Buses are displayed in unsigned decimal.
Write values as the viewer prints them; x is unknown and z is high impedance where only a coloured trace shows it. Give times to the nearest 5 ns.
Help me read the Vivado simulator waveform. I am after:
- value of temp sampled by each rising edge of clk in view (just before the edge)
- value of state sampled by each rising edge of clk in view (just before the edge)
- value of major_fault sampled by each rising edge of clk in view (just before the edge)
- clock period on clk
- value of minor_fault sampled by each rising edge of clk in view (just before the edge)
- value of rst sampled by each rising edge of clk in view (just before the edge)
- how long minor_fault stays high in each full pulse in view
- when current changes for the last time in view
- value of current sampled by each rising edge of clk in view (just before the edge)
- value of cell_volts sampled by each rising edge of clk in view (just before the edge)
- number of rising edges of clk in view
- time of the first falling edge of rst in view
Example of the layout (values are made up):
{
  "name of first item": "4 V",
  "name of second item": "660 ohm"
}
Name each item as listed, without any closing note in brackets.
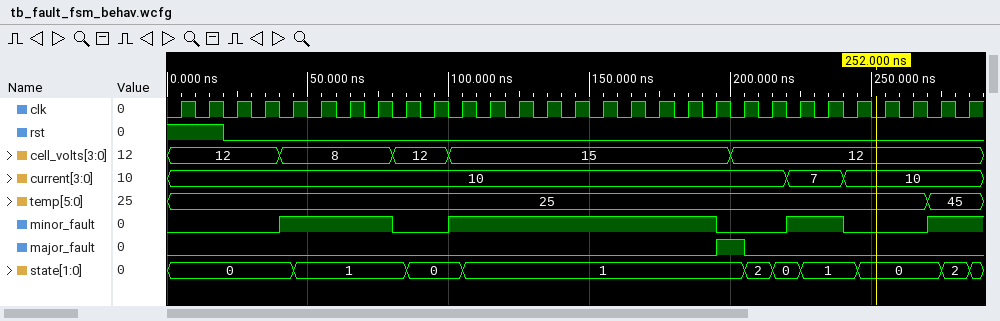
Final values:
{
  "value of temp sampled by each rising edge of clk in view": "25, 25, 25, 25, 25, 25, 25, 25, 25, 25, 25, 25, 25, 25, 25, 25, 25, 25, 25, 25, 25, 25, 25, 25, 25, 25, 25, 45, 45",
  "value of state sampled by each rising edge of clk in view": "0, 0, 0, 0, 0, 1, 1, 1, 1, 0, 0, 1, 1, 1, 1, 1, 1, 1, 1, 1, 1, 2, 0, 1, 1, 0, 0, 0, 2",
  "value of major_fault sampled by each rising edge of clk in view": "0 0 0 0 0 0 0 0 0 0 0 0 0 0 0 0 0 0 0 0 1 0 0 0 0 0 0 0 0",
  "clock period on clk": "10 ns",
  "value of minor_fault sampled by each rising edge of clk in view": "0 0 0 0 1 1 1 1 0 0 1 1 1 1 1 1 1 1 1 1 0 0 1 1 0 0 0 1 1",
  "value of rst sampled by each rising edge of clk in view": "1 1 0 0 0 0 0 0 0 0 0 0 0 0 0 0 0 0 0 0 0 0 0 0 0 0 0 0 0",
  "how long minor_fault stays high in each full pulse in view": "40 ns, 95 ns, 20 ns",
  "when current changes for the last time in view": "240 ns",
  "value of current sampled by each rising edge of clk in view": "10, 10, 10, 10, 10, 10, 10, 10, 10, 10, 10, 10, 10, 10, 10, 10, 10, 10, 10, 10, 10, 10, 7, 7, 10, 10, 10, 10, 10",
  "value of cell_volts sampled by each rising edge of clk in view": "12, 12, 12, 12, 8, 8, 8, 8, 12, 12, 15, 15, 15, 15, 15, 15, 15, 15, 15, 15, 12, 12, 12, 12, 12, 12, 12, 12, 12",
  "number of rising edges of clk in view": "29",
  "time of the first falling edge of rst in view": "20 ns"
}
